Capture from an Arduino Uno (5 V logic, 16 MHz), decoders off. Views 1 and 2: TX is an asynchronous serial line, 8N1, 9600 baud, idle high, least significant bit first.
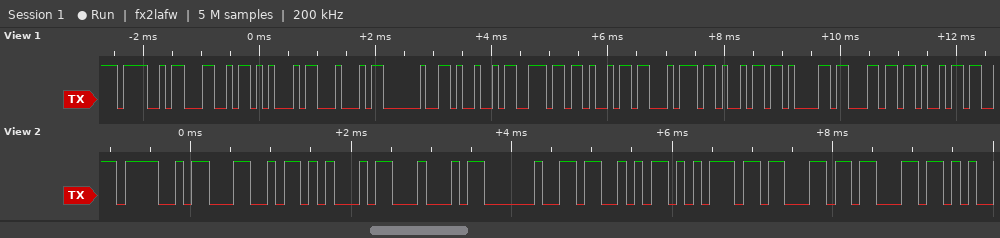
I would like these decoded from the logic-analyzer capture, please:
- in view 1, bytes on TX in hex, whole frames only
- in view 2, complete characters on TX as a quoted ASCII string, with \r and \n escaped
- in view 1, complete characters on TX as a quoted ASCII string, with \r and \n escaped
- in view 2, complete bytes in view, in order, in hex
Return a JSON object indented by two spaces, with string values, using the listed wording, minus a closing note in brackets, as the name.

{
  "in view 1, bytes on TX in hex, whole frames only": "4F 4C 45 44 20 49 6E 69 74 69 61 6C 69",
  "in view 2, complete characters on TX as a quoted ASCII string, with \\r and \\n escaped": "\"OLED Succ\"",
  "in view 1, complete characters on TX as a quoted ASCII string, with \\r and \\n escaped": "\"OLED Initiali\"",
  "in view 2, complete bytes in view, in order, in hex": "0x4F 0x4C 0x45 0x44 0x20 0x53 0x75 0x63 0x63"
}
